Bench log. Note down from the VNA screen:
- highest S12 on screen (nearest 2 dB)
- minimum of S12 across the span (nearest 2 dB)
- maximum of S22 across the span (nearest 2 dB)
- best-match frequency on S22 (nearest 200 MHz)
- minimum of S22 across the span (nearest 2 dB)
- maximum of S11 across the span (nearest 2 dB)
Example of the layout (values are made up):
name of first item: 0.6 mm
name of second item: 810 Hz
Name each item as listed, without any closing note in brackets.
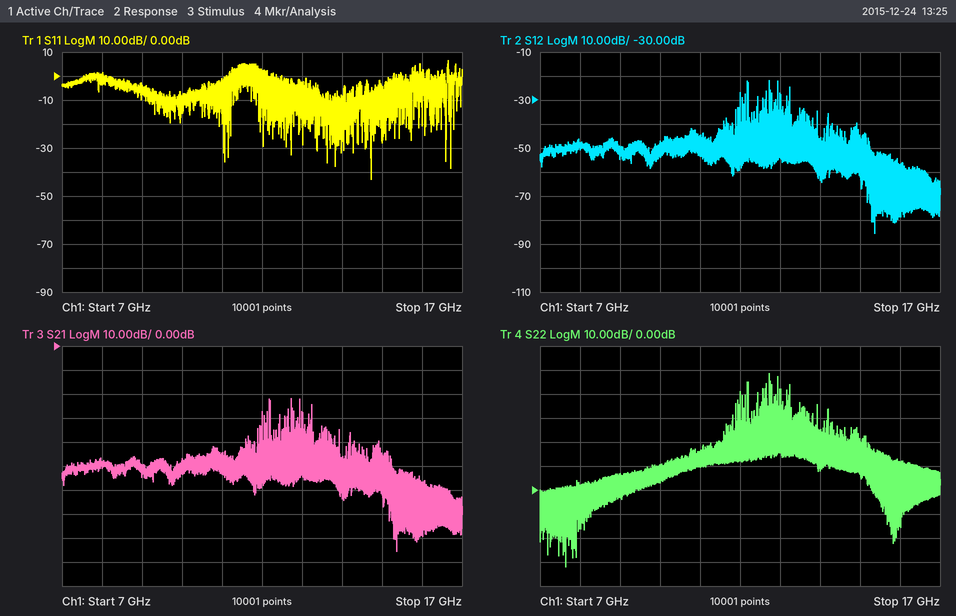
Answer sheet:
highest S12 on screen: -22 dB
minimum of S12 across the span: -86 dB
maximum of S22 across the span: 48 dB
best-match frequency on S22: 7.6 GHz
minimum of S22 across the span: -32 dB
maximum of S11 across the span: 6 dB
